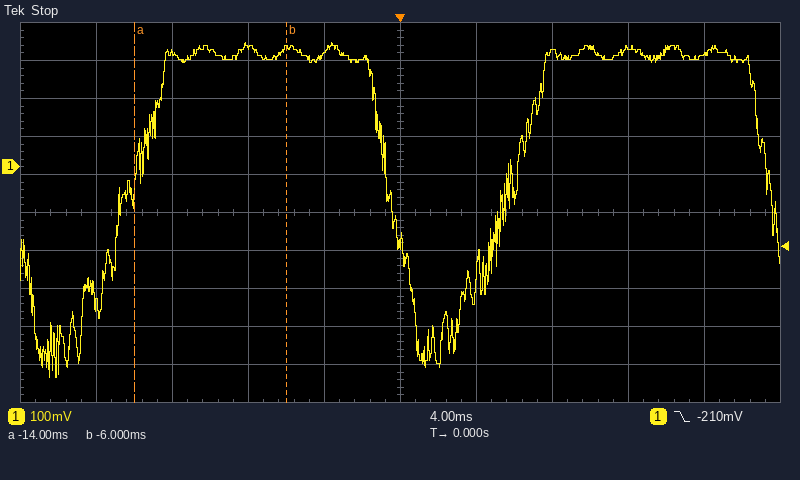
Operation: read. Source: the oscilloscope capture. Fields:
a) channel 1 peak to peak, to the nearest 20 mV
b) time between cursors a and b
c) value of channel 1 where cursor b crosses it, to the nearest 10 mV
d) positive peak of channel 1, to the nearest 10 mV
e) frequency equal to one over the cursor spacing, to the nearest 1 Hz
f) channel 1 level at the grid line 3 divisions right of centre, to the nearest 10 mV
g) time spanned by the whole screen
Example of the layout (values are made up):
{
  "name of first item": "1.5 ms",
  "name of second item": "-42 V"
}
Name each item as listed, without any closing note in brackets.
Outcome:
{
  "channel 1 peak to peak, to the nearest 20 mV": "880 mV",
  "time between cursors a and b": "8.0 ms",
  "value of channel 1 where cursor b crosses it, to the nearest 10 mV": "310 mV",
  "positive peak of channel 1, to the nearest 10 mV": "330 mV",
  "frequency equal to one over the cursor spacing, to the nearest 1 Hz": "125 Hz",
  "channel 1 level at the grid line 3 divisions right of centre, to the nearest 10 mV": "310 mV",
  "time spanned by the whole screen": "40 ms"
}
